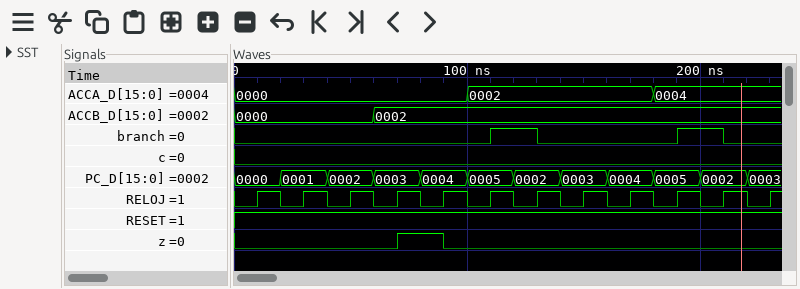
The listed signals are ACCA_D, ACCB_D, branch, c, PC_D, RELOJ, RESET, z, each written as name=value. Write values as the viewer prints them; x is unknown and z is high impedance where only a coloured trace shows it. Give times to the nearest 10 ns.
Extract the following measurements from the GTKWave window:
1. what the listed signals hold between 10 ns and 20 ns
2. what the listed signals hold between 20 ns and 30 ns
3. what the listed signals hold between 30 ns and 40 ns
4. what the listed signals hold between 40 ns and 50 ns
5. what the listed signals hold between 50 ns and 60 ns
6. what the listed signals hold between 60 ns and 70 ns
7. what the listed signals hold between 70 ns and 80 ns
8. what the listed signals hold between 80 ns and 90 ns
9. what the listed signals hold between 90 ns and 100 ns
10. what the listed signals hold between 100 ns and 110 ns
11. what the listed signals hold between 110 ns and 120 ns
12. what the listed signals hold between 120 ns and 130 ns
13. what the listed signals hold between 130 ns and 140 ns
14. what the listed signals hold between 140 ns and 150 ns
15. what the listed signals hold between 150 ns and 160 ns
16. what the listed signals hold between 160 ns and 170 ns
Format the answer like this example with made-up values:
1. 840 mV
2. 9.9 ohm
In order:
1. ACCA_D=0000, ACCB_D=0000, branch=0, c=0, PC_D=0000, RELOJ=1, RESET=1, z=0
2. ACCA_D=0000, ACCB_D=0000, branch=0, c=0, PC_D=0001, RELOJ=0, RESET=1, z=0
3. ACCA_D=0000, ACCB_D=0000, branch=0, c=0, PC_D=0001, RELOJ=1, RESET=1, z=0
4. ACCA_D=0000, ACCB_D=0000, branch=0, c=0, PC_D=0002, RELOJ=0, RESET=1, z=0
5. ACCA_D=0000, ACCB_D=0000, branch=0, c=0, PC_D=0002, RELOJ=1, RESET=1, z=0
6. ACCA_D=0000, ACCB_D=0002, branch=0, c=0, PC_D=0003, RELOJ=0, RESET=1, z=0
7. ACCA_D=0000, ACCB_D=0002, branch=0, c=0, PC_D=0003, RELOJ=1, RESET=1, z=1
8. ACCA_D=0000, ACCB_D=0002, branch=0, c=0, PC_D=0004, RELOJ=0, RESET=1, z=1
9. ACCA_D=0000, ACCB_D=0002, branch=0, c=0, PC_D=0004, RELOJ=1, RESET=1, z=0
10. ACCA_D=0002, ACCB_D=0002, branch=0, c=0, PC_D=0005, RELOJ=0, RESET=1, z=0
11. ACCA_D=0002, ACCB_D=0002, branch=1, c=0, PC_D=0005, RELOJ=1, RESET=1, z=0
12. ACCA_D=0002, ACCB_D=0002, branch=1, c=0, PC_D=0002, RELOJ=0, RESET=1, z=0
13. ACCA_D=0002, ACCB_D=0002, branch=0, c=0, PC_D=0002, RELOJ=1, RESET=1, z=0
14. ACCA_D=0002, ACCB_D=0002, branch=0, c=0, PC_D=0003, RELOJ=0, RESET=1, z=0
15. ACCA_D=0002, ACCB_D=0002, branch=0, c=0, PC_D=0003, RELOJ=1, RESET=1, z=0
16. ACCA_D=0002, ACCB_D=0002, branch=0, c=0, PC_D=0004, RELOJ=0, RESET=1, z=0
